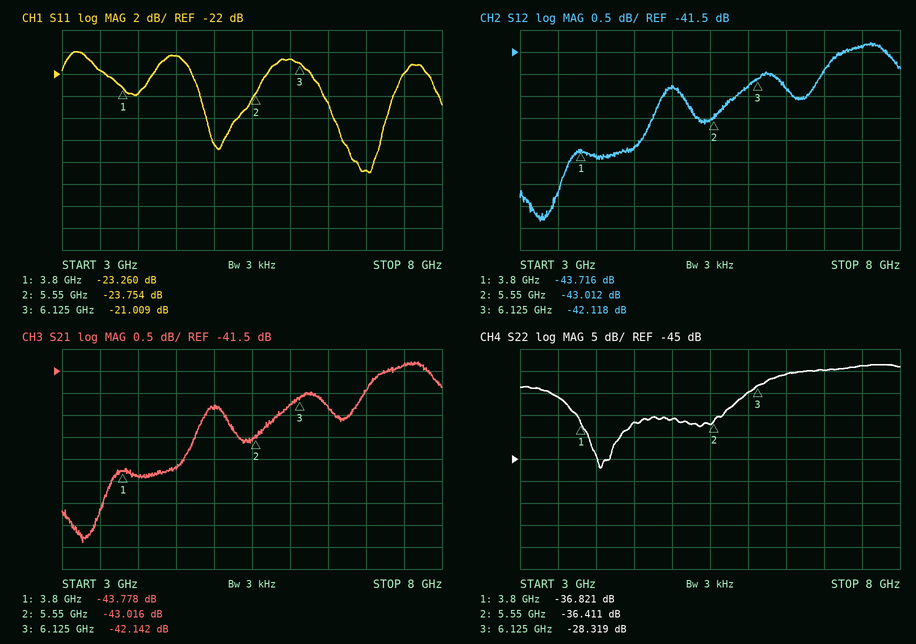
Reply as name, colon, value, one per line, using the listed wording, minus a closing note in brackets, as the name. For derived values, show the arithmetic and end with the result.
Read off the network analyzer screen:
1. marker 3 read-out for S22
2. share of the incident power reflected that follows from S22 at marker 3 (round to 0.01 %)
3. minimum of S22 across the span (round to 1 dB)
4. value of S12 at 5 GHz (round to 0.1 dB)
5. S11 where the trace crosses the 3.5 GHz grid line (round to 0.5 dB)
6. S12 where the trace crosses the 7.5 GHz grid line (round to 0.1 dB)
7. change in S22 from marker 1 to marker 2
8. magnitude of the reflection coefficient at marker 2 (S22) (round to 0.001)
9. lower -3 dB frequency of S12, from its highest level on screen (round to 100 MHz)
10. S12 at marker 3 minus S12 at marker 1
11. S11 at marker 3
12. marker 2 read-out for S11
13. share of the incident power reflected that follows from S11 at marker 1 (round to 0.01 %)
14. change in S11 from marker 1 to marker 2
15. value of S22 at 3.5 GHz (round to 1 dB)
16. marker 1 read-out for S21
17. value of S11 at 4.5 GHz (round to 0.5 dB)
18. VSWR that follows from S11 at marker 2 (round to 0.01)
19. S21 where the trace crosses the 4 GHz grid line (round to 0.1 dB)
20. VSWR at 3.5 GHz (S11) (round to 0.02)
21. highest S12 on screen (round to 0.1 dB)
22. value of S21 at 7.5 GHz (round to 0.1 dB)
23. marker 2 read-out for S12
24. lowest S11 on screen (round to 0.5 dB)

marker 3 read-out for S22: -28.319 dB
share of the incident power reflected that follows from S22 at marker 3: 10^(-28.319/10) ≈ 0.15 %
minimum of S22 across the span: -47 dB
value of S12 at 5 GHz: -42.3 dB
S11 where the trace crosses the 3.5 GHz grid line: -21.5 dB
S12 where the trace crosses the 7.5 GHz grid line: -41.4 dB
change in S22 from marker 1 to marker 2: -36.411 − (-36.821) = 0.410 dB
magnitude of the reflection coefficient at marker 2 (S22): 10^(-36.411/20) ≈ 0.015
lower -3 dB frequency of S12, from its highest level on screen: 3.6 GHz
S12 at marker 3 minus S12 at marker 1: -42.118 − (-43.716) = 1.598 dB
S11 at marker 3: -21.009 dB
marker 2 read-out for S11: -23.754 dB
share of the incident power reflected that follows from S11 at marker 1: 10^(-23.26/10) ≈ 0.47 %
change in S11 from marker 1 to marker 2: -23.754 − (-23.26) = -0.494 dB
value of S22 at 3.5 GHz: -31 dB
marker 1 read-out for S21: -43.778 dB
value of S11 at 4.5 GHz: -20.5 dB
VSWR that follows from S11 at marker 2: (1 + 0.0649)/(1 − 0.0649) ≈ 1.14
S21 where the trace crosses the 4 GHz grid line: -43.9 dB
VSWR at 3.5 GHz (S11): |Γ| = 10^(-21.5/20) = 0.0841; VSWR = (1 + 0.0841)/(1 − 0.0841) ≈ 1.18
highest S12 on screen: -41.3 dB
value of S21 at 7.5 GHz: -41.3 dB
marker 2 read-out for S12: -43.012 dB
lowest S11 on screen: -31.0 dB
